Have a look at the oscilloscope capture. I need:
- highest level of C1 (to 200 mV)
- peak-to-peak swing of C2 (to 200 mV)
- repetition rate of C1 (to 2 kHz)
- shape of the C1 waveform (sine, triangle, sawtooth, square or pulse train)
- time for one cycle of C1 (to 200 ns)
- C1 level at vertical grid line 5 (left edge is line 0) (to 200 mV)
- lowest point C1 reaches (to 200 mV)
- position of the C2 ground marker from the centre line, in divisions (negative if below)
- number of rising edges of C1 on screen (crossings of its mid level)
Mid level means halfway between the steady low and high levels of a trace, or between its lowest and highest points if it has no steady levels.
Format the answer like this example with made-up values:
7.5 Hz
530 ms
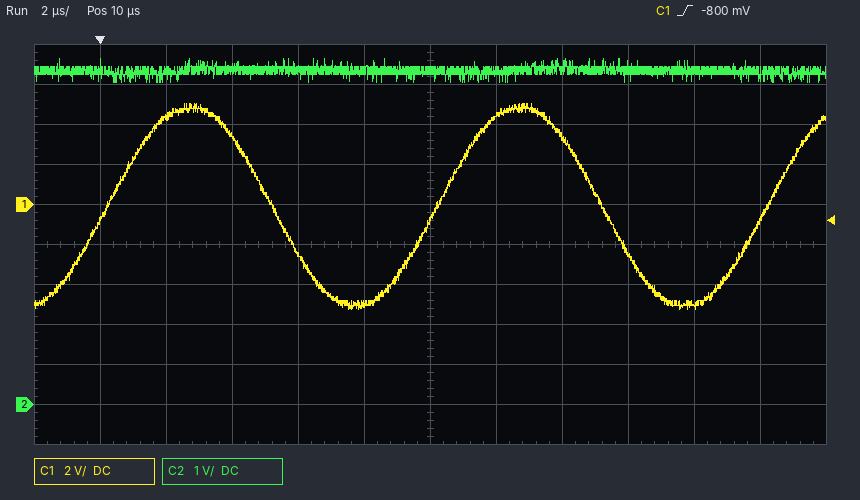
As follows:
5.0 V
600 mV
100 kHz
sine
10.0 µs
-5.0 V
-5.2 V
-4.0 div
3
